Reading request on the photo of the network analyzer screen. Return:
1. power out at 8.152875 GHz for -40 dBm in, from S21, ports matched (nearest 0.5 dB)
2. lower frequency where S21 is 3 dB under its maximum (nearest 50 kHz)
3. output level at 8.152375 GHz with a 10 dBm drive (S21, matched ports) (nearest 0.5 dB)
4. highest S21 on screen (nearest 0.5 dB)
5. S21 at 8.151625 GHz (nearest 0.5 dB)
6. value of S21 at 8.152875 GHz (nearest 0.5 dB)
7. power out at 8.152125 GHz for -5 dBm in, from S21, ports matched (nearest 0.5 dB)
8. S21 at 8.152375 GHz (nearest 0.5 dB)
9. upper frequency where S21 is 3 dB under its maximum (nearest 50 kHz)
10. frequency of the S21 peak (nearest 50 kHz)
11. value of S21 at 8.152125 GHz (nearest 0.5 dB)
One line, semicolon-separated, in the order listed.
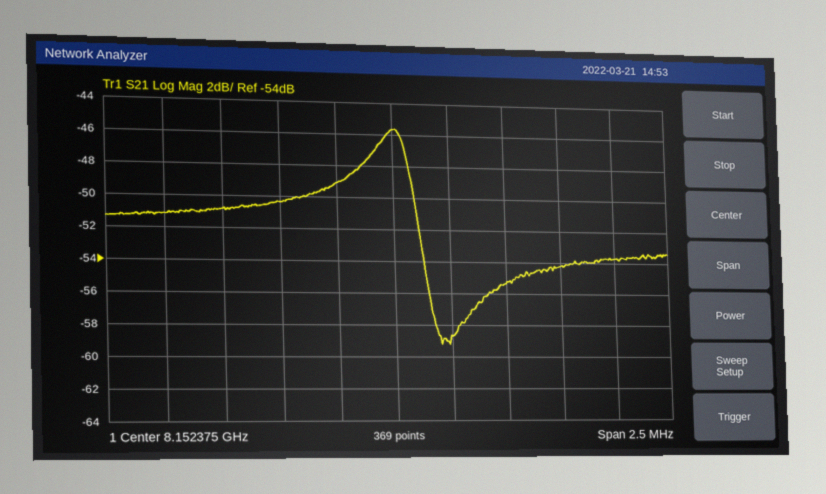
-95.5 dBm; 8.15220 GHz; -35.5 dBm; -45.5 dB; -51.0 dB; -55.5 dB; -54.0 dBm; -45.5 dB; 8.15245 GHz; 8.15240 GHz; -49.0 dB
